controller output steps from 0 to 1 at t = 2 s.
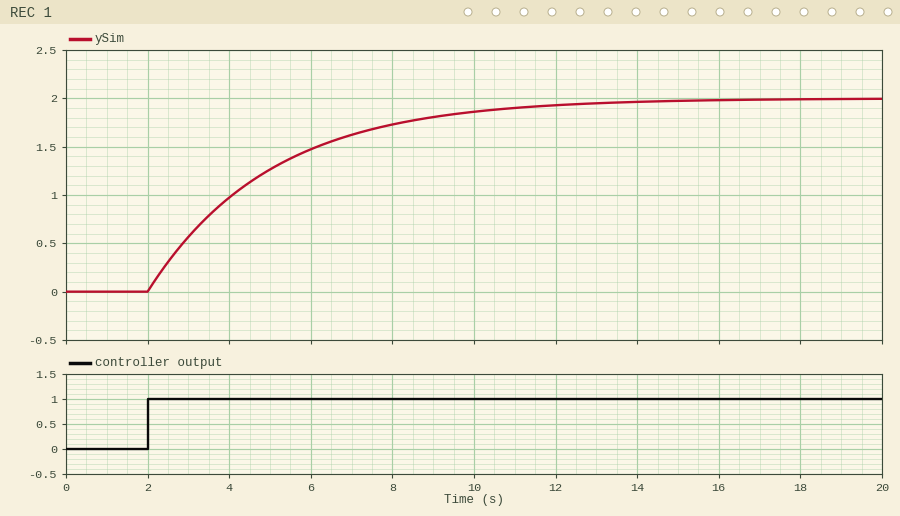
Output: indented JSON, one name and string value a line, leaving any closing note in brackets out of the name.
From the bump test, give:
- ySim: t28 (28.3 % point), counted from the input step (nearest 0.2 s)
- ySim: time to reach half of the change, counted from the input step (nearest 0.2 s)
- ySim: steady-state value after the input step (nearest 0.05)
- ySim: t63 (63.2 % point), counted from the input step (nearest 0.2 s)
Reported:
{
  "ySim: t28 (28.3 % point), counted from the input step": "1.0 s",
  "ySim: time to reach half of the change, counted from the input step": "2.0 s",
  "ySim: steady-state value after the input step": "2.00",
  "ySim: t63 (63.2 % point), counted from the input step": "3.0 s"
}
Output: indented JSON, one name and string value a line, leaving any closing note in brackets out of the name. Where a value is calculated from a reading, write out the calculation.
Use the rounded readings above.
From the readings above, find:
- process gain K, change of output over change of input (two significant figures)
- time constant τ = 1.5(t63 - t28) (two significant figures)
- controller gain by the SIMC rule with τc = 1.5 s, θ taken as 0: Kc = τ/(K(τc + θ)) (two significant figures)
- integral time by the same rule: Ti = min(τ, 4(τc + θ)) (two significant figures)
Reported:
{
  "process gain K, change of output over change of input": "(2 - 0) / 1 = 2.0",
  "time constant τ = 1.5(t63 - t28)": "1.5 × (3 - 1) = 3.0 s",
  "controller gain by the SIMC rule with τc = 1.5 s, θ taken as 0: Kc = τ/(K(τc + θ))": "3 / (2 × (1.5 + 0)) = 1.0",
  "integral time by the same rule: Ti = min(τ, 4(τc + θ))": "min(3, 4 × (1.5 + 0)) = 3.0 s"
}
